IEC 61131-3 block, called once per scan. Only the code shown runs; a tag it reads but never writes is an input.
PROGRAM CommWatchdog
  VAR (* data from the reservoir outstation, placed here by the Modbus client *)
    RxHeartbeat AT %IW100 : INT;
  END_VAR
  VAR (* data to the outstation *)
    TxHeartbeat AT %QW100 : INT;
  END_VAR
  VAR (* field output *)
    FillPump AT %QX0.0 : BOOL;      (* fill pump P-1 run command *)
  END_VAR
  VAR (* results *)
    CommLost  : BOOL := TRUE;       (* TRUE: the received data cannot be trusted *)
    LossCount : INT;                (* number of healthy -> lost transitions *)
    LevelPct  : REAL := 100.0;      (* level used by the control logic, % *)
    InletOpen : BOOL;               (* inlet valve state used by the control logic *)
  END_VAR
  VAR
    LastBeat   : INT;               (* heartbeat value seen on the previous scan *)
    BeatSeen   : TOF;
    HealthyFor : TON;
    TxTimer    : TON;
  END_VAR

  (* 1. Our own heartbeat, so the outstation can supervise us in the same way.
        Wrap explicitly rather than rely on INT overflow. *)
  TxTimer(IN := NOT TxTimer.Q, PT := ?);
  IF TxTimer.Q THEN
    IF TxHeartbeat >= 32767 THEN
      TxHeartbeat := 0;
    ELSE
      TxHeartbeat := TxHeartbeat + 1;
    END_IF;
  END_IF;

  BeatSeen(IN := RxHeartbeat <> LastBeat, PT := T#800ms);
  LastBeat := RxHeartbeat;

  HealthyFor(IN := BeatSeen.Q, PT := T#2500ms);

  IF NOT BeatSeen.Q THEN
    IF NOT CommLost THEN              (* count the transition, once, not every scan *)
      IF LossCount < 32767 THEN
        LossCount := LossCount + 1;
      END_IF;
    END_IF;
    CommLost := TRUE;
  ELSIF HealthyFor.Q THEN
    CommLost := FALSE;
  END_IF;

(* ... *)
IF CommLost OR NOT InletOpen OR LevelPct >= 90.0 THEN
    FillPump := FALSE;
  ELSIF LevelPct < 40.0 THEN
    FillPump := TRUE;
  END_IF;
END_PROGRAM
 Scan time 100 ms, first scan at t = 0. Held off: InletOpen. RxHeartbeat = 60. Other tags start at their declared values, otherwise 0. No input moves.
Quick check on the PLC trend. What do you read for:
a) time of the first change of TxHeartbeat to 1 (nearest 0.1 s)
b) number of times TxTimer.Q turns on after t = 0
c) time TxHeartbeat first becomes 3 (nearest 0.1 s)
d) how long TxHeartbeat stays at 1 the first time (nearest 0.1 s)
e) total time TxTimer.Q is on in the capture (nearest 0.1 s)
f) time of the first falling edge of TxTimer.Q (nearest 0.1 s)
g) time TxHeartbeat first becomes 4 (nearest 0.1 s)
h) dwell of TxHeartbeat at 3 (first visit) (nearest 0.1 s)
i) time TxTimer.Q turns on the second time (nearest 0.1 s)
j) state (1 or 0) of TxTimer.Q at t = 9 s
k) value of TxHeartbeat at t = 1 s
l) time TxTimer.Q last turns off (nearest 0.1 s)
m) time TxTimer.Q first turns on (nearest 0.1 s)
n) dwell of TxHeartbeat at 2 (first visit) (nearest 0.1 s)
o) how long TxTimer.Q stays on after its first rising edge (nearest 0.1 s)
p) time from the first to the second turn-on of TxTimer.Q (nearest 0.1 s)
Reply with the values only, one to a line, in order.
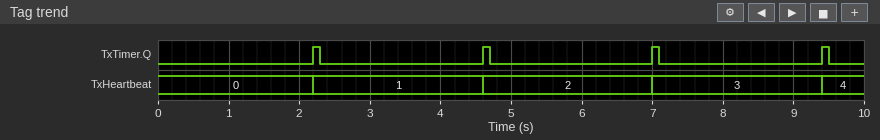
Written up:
2.2 s
4
7.0 s
2.4 s
0.4 s
2.3 s
9.4 s
2.4 s
4.6 s
0
0
9.5 s
2.2 s
2.4 s
0.1 s
2.4 s
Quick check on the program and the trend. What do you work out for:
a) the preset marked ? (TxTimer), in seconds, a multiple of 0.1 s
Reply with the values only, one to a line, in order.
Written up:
2.2 s
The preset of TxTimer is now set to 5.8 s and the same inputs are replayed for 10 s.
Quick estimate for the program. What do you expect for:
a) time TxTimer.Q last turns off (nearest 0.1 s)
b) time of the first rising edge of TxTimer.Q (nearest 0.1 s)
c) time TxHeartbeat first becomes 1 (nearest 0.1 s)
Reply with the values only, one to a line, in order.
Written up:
5.9 s
5.8 s
5.8 s
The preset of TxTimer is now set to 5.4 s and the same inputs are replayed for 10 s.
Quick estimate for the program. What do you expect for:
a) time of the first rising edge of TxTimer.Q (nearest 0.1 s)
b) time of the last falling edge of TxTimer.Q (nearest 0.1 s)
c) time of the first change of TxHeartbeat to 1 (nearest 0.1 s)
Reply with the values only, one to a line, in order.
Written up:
5.4 s
5.5 s
5.4 s
